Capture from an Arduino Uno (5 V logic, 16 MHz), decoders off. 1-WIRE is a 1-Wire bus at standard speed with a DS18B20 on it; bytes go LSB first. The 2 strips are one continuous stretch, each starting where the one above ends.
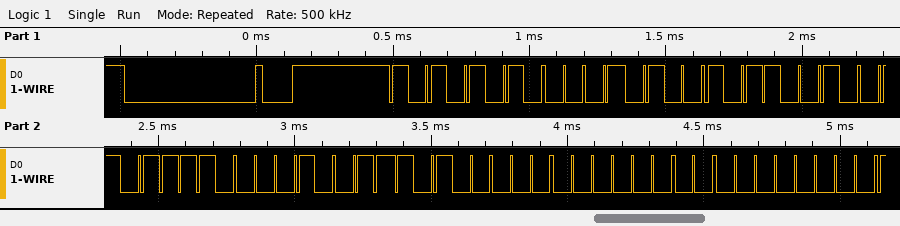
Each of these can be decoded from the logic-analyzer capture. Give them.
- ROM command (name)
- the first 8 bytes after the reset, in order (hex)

Match ROM
55 28 4D 7A C8 05 00 00
